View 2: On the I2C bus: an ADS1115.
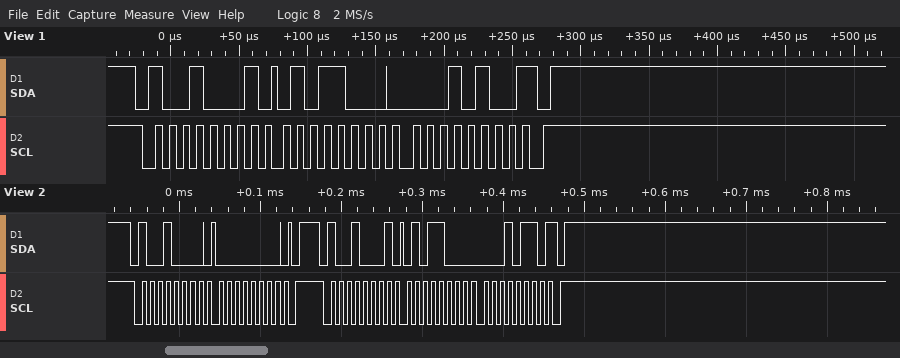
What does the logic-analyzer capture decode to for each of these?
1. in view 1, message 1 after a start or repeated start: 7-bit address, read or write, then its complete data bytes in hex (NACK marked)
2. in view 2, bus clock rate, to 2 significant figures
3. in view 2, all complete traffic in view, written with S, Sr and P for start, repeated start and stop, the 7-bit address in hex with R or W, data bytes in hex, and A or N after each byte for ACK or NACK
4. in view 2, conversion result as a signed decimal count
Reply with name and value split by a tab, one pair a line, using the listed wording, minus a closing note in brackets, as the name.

in view 1, message 1 after a start or repeated start: 7-bit address, read or write, then its complete data bytes in hex	0x48 read: 58 14 NACK
in view 2, bus clock rate, to 2 significant figures	100 kHz
in view 2, all complete traffic in view, written with S, Sr and P for start, repeated start and stop, the 7-bit address in hex with R or W, data bytes in hex, and A or N after each byte for ACK or NACK	S 48W A 00 A P S 48R A 58 A 16 N P
in view 2, conversion result as a signed decimal count	22550
